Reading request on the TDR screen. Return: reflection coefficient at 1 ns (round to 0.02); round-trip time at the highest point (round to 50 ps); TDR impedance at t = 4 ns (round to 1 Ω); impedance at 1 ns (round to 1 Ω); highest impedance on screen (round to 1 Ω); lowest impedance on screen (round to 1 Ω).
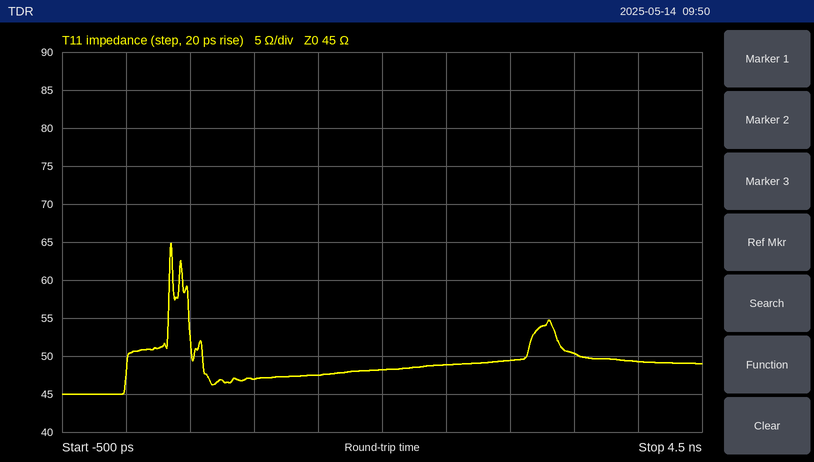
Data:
+0.02
350 ps
49 Ω
47 Ω
65 Ω
45 Ω
